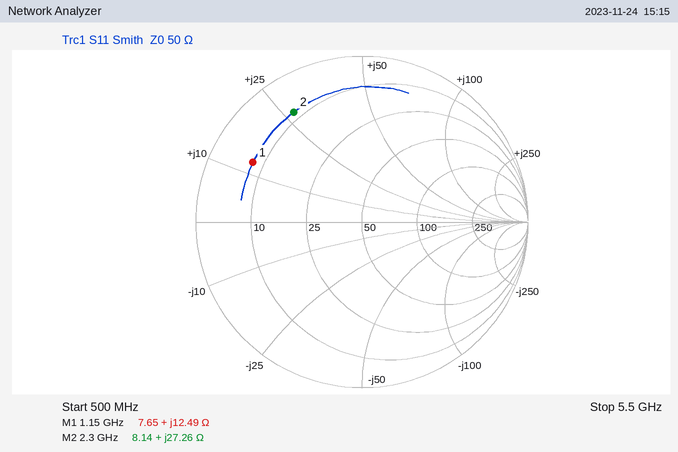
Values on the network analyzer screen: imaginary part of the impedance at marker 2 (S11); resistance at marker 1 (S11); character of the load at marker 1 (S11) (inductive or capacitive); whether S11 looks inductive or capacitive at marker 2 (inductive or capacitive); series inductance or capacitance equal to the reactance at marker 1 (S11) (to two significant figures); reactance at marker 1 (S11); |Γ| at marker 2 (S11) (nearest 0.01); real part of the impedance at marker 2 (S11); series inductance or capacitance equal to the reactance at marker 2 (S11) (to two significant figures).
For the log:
+27.26 Ω
7.65 Ω
inductive
inductive
1.7 nH
+12.49 Ω
0.78
8.14 Ω
1.9 nH
